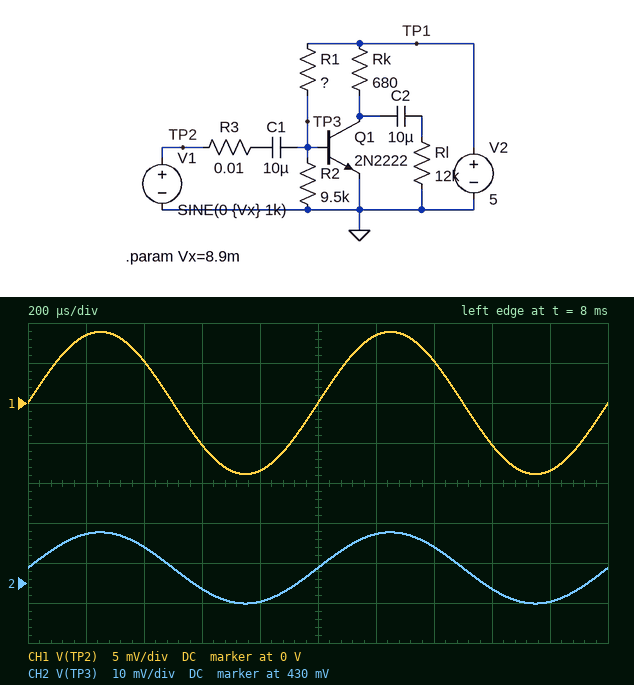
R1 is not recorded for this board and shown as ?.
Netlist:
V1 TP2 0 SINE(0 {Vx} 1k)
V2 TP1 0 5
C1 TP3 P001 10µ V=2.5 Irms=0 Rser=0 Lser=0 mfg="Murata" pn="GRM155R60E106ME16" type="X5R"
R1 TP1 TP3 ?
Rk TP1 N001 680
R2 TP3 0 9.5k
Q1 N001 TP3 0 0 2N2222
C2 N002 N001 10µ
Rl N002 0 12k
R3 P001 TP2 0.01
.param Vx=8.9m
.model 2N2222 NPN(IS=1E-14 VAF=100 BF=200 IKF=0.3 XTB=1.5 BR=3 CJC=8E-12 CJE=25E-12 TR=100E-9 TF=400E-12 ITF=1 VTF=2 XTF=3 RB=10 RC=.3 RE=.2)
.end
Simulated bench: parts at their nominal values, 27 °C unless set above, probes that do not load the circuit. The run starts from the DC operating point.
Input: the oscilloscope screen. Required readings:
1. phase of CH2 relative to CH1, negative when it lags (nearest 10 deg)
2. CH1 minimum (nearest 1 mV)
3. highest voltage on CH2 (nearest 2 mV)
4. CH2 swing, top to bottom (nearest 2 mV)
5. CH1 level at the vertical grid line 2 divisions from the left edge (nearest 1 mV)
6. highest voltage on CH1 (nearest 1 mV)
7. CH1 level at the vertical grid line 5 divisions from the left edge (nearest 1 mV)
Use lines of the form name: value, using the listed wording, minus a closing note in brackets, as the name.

phase of CH2 relative to CH1, negative when it lags: 0 deg
CH1 minimum: -9 mV
highest voltage on CH2: 442 mV
CH2 swing, top to bottom: 18 mV
CH1 level at the vertical grid line 2 divisions from the left edge: 5 mV
highest voltage on CH1: 9 mV
CH1 level at the vertical grid line 5 divisions from the left edge: 0 V
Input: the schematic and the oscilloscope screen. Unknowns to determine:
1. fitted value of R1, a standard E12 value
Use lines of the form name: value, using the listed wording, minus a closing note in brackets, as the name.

fitted value of R1, a standard E12 value: 100 kΩ
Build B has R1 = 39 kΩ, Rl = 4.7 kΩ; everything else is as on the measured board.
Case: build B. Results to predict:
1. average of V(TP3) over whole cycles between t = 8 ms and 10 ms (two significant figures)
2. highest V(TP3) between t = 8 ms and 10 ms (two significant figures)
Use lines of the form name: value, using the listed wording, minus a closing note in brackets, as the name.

average of V(TP3) over whole cycles between t = 8 ms and 10 ms: 700 mV
highest V(TP3) between t = 8 ms and 10 ms: 710 mV
